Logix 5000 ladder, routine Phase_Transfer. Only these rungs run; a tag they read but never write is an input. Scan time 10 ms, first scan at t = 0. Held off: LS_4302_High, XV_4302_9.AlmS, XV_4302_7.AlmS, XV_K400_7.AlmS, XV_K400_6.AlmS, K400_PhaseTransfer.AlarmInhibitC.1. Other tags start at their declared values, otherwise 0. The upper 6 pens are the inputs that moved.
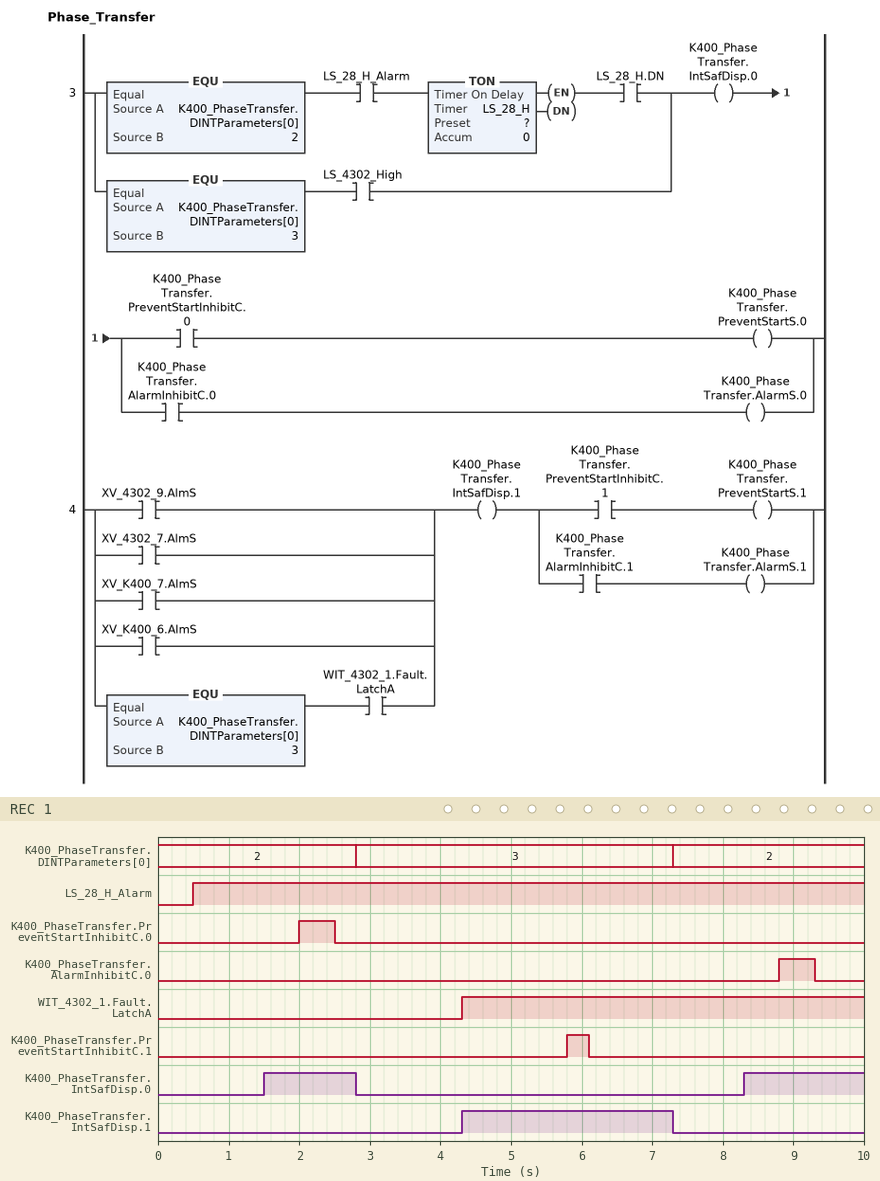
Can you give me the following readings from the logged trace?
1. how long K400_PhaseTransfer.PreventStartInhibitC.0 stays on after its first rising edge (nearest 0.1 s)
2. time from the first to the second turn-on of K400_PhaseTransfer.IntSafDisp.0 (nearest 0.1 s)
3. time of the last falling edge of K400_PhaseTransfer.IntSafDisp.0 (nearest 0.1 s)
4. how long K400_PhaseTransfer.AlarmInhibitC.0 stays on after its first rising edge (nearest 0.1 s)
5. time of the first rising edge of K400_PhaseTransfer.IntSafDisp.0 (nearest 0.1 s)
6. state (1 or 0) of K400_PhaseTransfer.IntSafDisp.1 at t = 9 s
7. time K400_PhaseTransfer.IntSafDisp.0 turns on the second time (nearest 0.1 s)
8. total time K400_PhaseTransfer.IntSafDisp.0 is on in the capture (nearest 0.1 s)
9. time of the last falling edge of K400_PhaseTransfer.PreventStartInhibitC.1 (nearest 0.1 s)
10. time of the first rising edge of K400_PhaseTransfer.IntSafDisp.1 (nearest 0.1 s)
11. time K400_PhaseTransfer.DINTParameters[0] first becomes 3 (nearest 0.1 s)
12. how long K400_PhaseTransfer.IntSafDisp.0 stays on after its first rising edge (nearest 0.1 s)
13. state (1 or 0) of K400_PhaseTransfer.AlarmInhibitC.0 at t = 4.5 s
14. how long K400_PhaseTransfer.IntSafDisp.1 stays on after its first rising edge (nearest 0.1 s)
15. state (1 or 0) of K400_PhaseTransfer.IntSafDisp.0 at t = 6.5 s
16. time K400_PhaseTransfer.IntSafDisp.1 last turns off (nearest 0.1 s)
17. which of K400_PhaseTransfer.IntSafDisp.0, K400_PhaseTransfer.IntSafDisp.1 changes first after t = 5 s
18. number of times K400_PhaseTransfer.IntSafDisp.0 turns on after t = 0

0.5 s
6.8 s
2.8 s
0.5 s
1.5 s
0
8.3 s
3.0 s
6.1 s
4.3 s
2.8 s
1.3 s
0
3.0 s
0
7.3 s
K400_PhaseTransfer.IntSafDisp.1
2
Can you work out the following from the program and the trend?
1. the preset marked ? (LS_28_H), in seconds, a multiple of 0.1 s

1.0 s
